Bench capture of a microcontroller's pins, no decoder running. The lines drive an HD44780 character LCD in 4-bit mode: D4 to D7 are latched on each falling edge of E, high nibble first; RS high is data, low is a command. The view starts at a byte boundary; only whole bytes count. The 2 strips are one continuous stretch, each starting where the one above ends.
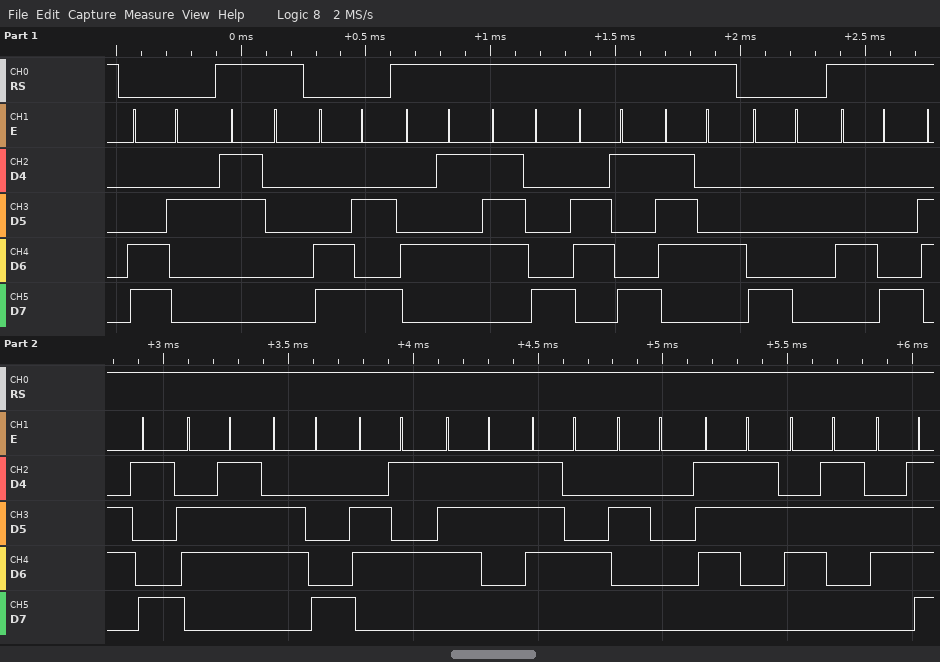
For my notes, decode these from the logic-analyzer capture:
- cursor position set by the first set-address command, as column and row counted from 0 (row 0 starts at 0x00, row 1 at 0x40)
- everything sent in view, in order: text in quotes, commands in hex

column 2, row 1
0xC2 "0" 0xCA "Exit" 0x80 "Highest sco"
